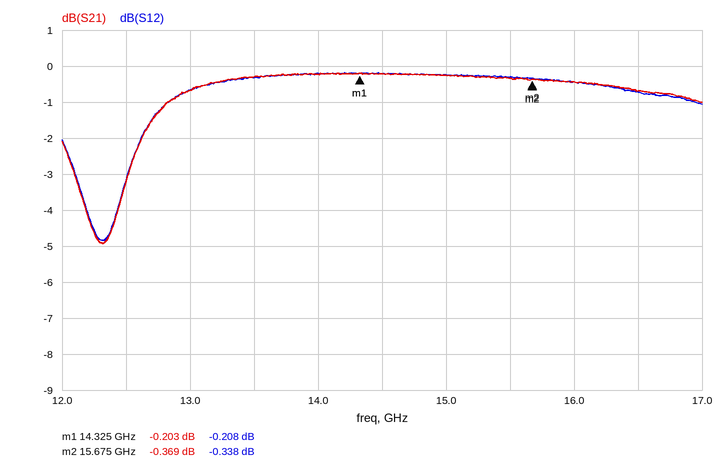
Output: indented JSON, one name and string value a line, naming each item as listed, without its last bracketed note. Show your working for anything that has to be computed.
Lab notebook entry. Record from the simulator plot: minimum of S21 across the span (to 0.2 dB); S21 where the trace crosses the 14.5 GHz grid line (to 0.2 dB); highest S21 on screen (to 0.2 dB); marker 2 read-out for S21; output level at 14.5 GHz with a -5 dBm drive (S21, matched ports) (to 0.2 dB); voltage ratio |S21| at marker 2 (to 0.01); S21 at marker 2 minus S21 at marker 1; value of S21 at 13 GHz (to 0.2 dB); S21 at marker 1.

{
  "minimum of S21 across the span": "-5.0 dB",
  "S21 where the trace crosses the 14.5 GHz grid line": "-0.2 dB",
  "highest S21 on screen": "-0.2 dB",
  "marker 2 read-out for S21": "-0.369 dB",
  "output level at 14.5 GHz with a -5 dBm drive (S21, matched ports)": "-5 dBm + (-0.2 dB) = -5.2 dBm",
  "voltage ratio |S21| at marker 2": "10^(-0.369/20) ≈ 0.96",
  "S21 at marker 2 minus S21 at marker 1": "-0.369 − (-0.203) = -0.166 dB",
  "value of S21 at 13 GHz": "-0.6 dB",
  "S21 at marker 1": "-0.203 dB"
}
